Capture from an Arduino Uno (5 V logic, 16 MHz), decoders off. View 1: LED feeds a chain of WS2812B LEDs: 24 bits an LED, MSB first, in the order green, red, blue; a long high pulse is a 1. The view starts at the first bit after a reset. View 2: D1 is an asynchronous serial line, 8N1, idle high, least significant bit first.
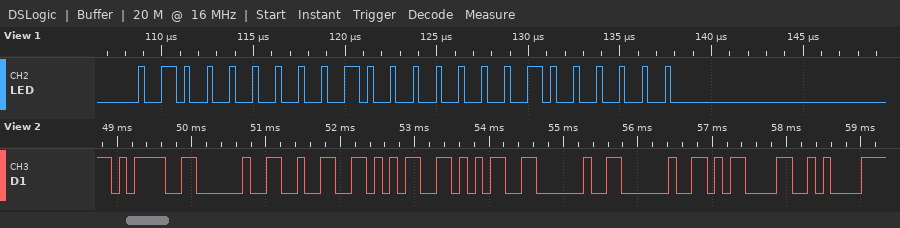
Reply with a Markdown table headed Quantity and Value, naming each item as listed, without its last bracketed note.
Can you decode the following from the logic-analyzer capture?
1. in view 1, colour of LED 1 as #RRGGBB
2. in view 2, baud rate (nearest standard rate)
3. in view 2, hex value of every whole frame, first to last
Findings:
| Quantity | Value |
|---|---|
| in view 1, colour of LED 1 as #RRGGBB | #404040 |
| in view 2, baud rate | 9600 baud |
| in view 2, hex value of every whole frame, first to last | 3D 20 32 35 35 20 20 0D 0A |
